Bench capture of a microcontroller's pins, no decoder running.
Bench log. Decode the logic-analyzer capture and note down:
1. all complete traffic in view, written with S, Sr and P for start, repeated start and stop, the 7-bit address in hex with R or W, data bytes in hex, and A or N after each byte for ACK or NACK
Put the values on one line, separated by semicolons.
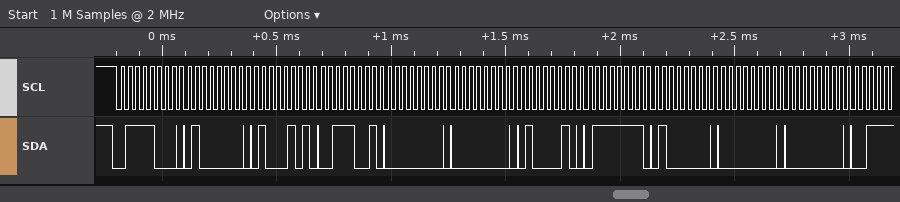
S 3CW A 40 A 45 A 39 A 00 A 00 A 42 A 7F A 40 A 00 A 00 A
